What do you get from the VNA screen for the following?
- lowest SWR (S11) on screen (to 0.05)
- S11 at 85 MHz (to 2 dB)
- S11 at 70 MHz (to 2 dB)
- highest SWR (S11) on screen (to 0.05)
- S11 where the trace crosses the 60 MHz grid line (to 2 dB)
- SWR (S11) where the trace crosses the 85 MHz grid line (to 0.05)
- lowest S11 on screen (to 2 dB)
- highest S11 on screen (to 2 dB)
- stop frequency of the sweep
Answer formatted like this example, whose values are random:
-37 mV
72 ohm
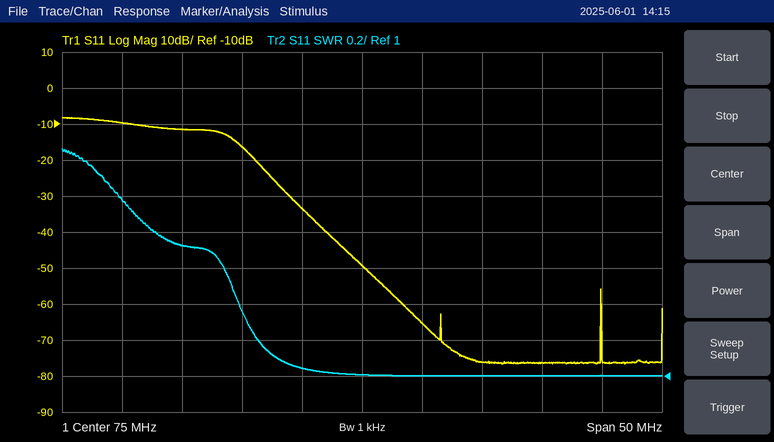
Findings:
1.00
-76 dB
-34 dB
2.25
-12 dB
1.00
-76 dB
-8 dB
100 MHz
